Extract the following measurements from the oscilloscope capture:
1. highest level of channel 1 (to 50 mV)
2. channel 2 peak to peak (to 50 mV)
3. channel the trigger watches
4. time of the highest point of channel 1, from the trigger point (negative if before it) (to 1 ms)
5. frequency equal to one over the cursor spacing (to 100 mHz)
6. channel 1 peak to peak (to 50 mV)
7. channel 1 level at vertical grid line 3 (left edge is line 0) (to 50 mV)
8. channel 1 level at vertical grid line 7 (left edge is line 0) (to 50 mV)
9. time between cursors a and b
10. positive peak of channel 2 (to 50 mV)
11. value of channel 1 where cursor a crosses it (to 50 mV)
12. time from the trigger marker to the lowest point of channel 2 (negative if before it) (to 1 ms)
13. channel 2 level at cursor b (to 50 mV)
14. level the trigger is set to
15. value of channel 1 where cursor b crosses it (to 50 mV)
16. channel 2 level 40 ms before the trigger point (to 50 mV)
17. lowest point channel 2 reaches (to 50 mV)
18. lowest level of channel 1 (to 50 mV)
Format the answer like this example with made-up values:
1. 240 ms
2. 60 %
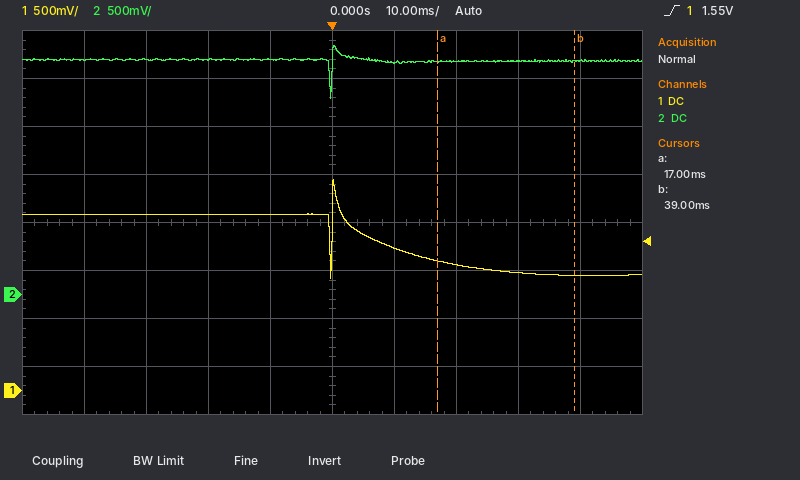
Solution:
1. 2.20 V
2. 550 mV
3. channel 1
4. 0 ms
5. 45.5 Hz
6. 1.05 V
7. 1.85 V
8. 1.30 V
9. 22 ms
10. 2.60 V
11. 1.35 V
12. 0 ms
13. 2.45 V
14. 1.55 V
15. 1.20 V
16. 2.45 V
17. 2.05 V
18. 1.15 V
